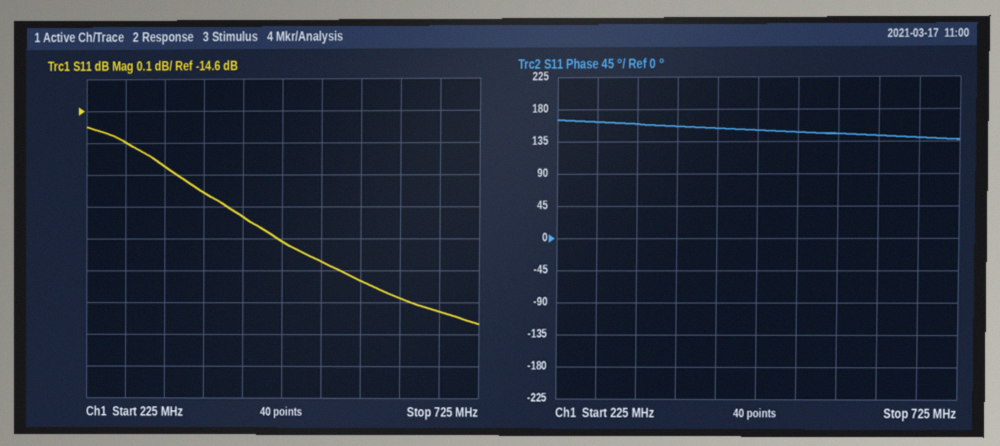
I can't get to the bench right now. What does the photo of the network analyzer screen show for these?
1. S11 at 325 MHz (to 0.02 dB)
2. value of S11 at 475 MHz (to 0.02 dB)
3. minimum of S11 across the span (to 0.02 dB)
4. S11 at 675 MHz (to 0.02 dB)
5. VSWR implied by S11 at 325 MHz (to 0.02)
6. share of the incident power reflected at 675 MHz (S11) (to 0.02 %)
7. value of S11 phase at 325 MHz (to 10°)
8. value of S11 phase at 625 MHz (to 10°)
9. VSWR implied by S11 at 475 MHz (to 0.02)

-14.78 dB
-15.00 dB
-15.26 dB
-15.22 dB
1.44
3.00 %
160°
140°
1.44
